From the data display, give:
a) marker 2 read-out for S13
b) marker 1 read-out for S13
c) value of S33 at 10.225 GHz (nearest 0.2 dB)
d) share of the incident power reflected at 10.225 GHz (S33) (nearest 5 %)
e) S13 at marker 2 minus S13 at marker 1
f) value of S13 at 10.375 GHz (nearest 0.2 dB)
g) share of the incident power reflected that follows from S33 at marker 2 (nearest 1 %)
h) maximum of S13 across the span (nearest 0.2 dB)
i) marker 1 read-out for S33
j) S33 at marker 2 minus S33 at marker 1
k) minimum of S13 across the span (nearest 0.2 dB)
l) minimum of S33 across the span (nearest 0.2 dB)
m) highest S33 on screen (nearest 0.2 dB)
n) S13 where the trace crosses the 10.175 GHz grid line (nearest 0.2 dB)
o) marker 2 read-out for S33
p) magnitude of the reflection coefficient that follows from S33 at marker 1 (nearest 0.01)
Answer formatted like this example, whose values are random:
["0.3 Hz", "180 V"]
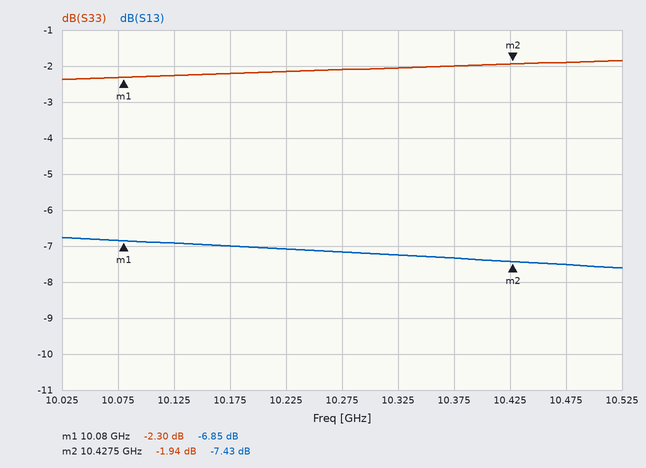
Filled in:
["-7.43 dB", "-6.85 dB", "-2.2 dB", "60 %", "-0.58 dB", "-7.4 dB", "64 %", "-6.8 dB", "-2.30 dB", "0.36 dB", "-7.6 dB", "-2.4 dB", "-1.8 dB", "-7.0 dB", "-1.94 dB", "0.77"]
